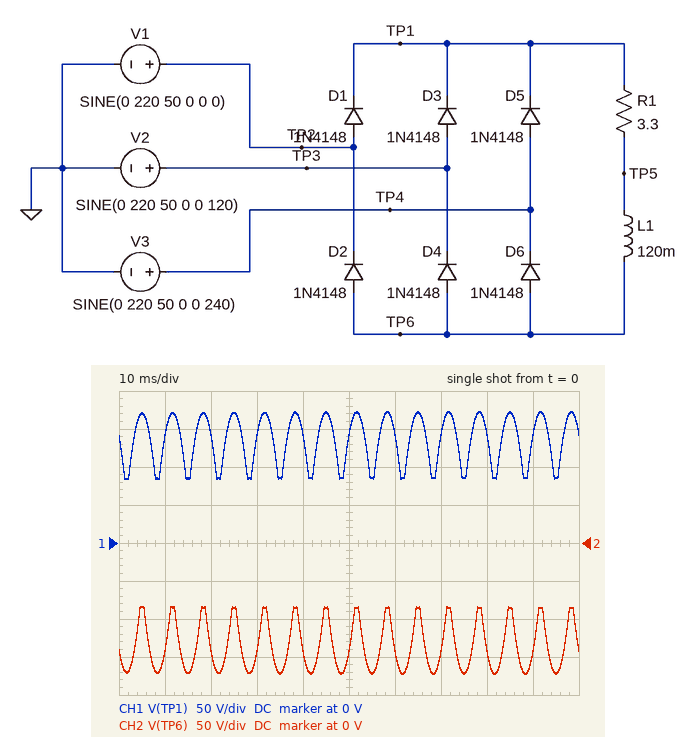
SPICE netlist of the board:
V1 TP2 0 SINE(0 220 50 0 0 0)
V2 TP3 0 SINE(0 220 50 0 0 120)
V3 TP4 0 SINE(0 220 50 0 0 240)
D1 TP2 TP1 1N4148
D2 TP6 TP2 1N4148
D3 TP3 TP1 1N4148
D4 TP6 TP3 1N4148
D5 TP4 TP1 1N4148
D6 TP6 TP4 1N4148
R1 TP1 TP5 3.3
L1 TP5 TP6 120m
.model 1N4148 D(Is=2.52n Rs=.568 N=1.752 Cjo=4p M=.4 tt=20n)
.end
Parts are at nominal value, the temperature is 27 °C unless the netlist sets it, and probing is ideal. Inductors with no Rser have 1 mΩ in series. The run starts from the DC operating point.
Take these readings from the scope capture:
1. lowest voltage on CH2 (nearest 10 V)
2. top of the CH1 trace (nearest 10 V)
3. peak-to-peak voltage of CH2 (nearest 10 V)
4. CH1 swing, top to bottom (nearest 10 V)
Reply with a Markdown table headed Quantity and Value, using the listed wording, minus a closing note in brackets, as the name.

| Quantity | Value |
|---|---|
| lowest voltage on CH2 | -170 V |
| top of the CH1 trace | 170 V |
| peak-to-peak voltage of CH2 | 90 V |
| CH1 swing, top to bottom | 90 V |
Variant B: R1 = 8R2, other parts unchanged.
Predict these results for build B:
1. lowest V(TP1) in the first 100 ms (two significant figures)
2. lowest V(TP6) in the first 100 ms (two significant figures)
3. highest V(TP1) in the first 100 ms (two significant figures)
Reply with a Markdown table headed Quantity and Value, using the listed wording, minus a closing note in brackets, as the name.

| Quantity | Value |
|---|---|
| lowest V(TP1) in the first 100 ms | 97 V |
| lowest V(TP6) in the first 100 ms | -200 V |
| highest V(TP1) in the first 100 ms | 200 V |
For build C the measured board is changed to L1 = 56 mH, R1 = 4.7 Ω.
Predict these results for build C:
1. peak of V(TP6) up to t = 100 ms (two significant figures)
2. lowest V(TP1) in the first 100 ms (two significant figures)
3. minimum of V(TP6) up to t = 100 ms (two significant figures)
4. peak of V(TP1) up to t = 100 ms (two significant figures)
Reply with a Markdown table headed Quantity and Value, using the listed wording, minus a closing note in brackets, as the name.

| Quantity | Value |
|---|---|
| peak of V(TP6) up to t = 100 ms | -90 V |
| lowest V(TP1) in the first 100 ms | 90 V |
| minimum of V(TP6) up to t = 100 ms | -180 V |
| peak of V(TP1) up to t = 100 ms | 180 V |
